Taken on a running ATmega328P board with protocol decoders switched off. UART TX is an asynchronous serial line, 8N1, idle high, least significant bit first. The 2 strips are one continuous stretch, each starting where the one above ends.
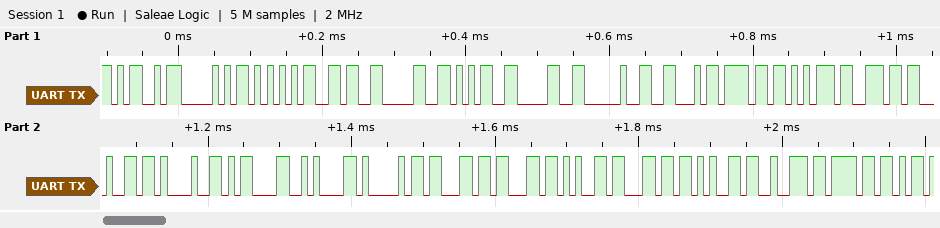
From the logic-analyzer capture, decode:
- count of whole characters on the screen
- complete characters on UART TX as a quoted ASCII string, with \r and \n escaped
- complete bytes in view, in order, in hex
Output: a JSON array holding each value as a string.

["24", "\"MPU6050 Found!\\r\\nAccelero\"", "0x4D 0x50 0x55 0x36 0x30 0x35 0x30 0x20 0x46 0x6F 0x75 0x6E 0x64 0x21 0x0D 0x0A 0x41 0x63 0x63 0x65 0x6C 0x65 0x72 0x6F"]
